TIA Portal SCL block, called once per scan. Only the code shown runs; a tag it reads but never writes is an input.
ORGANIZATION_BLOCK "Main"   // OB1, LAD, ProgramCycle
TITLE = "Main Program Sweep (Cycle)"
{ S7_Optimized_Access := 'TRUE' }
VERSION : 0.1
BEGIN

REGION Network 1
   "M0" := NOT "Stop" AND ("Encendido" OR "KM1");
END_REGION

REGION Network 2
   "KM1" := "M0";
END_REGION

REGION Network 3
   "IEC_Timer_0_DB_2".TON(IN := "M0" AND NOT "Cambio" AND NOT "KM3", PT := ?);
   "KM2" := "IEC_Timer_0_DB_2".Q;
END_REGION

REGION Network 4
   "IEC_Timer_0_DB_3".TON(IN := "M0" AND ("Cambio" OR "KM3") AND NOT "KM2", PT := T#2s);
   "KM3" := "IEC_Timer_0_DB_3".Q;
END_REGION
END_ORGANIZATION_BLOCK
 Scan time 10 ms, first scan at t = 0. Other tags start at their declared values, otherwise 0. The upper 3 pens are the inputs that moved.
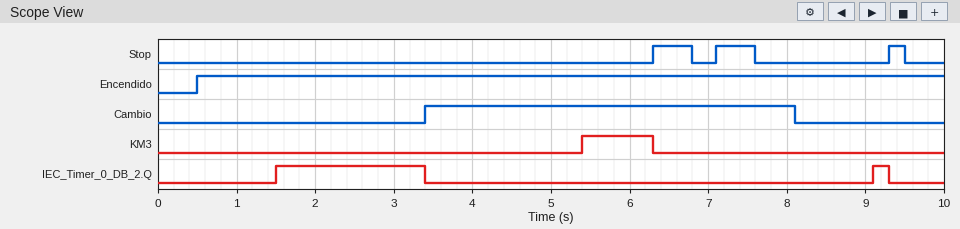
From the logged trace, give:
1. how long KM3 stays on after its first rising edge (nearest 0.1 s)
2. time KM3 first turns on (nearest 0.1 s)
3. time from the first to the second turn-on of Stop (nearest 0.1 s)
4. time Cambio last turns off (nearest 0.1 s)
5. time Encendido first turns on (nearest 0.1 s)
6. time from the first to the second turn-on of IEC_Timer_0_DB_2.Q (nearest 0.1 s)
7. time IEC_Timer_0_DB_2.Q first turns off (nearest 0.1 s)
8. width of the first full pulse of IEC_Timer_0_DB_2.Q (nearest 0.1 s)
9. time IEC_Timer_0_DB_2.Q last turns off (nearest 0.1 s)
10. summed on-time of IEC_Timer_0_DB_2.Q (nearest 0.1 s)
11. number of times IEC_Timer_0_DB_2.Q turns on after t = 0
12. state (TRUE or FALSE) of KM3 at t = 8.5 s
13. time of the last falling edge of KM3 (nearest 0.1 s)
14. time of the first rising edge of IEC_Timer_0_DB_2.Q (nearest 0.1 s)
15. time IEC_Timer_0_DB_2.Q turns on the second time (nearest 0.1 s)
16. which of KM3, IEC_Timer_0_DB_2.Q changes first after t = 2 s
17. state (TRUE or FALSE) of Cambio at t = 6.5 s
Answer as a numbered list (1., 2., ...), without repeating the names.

1. 0.9 s
2. 5.4 s
3. 0.8 s
4. 8.1 s
5. 0.5 s
6. 7.6 s
7. 3.4 s
8. 1.9 s
9. 9.3 s
10. 2.1 s
11. 2
12. FALSE
13. 6.3 s
14. 1.5 s
15. 9.1 s
16. IEC_Timer_0_DB_2.Q
17. TRUE
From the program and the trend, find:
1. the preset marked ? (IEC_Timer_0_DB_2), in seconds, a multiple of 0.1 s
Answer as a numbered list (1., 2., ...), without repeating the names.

1. 1.0 s
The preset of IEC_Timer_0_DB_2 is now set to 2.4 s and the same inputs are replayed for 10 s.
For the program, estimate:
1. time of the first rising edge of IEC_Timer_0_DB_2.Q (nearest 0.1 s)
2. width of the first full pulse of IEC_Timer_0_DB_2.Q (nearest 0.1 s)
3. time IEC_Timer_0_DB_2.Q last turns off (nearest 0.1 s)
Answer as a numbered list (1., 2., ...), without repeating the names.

1. 2.9 s
2. 0.5 s
3. 3.4 s
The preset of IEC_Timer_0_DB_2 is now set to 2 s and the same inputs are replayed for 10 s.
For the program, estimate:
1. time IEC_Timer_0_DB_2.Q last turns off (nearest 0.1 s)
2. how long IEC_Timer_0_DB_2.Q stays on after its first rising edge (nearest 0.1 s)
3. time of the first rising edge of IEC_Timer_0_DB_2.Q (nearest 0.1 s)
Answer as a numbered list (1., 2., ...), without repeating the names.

1. 3.4 s
2. 0.9 s
3. 2.5 s
